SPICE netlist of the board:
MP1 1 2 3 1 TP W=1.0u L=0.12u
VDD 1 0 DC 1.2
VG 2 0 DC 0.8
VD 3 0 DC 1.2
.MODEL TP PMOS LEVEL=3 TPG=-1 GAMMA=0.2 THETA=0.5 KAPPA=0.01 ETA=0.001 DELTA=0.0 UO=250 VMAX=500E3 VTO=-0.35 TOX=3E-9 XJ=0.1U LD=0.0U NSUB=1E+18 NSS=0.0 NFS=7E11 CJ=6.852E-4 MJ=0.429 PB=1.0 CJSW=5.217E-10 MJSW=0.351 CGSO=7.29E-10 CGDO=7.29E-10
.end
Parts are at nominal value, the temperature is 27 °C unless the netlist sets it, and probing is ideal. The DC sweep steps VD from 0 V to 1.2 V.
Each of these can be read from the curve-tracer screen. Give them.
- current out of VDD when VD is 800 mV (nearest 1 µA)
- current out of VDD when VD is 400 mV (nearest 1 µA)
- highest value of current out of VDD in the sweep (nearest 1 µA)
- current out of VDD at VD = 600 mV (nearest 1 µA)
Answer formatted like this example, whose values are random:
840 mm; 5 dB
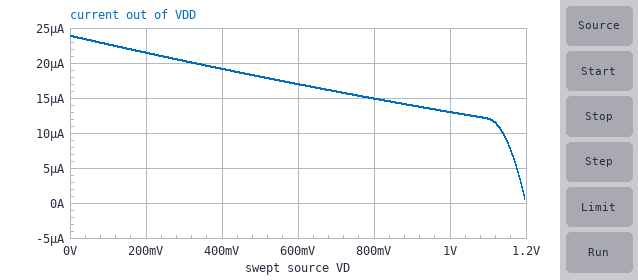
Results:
15 µA; 19 µA; 24 µA; 17 µA
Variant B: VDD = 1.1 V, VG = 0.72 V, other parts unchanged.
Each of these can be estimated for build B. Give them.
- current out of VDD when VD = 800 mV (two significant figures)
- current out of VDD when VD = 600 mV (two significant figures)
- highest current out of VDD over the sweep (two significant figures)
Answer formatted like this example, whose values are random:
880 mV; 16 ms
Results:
9.7 µA; 11 µA; 17 µA
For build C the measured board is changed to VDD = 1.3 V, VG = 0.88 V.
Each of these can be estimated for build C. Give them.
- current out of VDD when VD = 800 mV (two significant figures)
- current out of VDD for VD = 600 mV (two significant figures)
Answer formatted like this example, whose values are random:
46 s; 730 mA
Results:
21 µA; 24 µA
